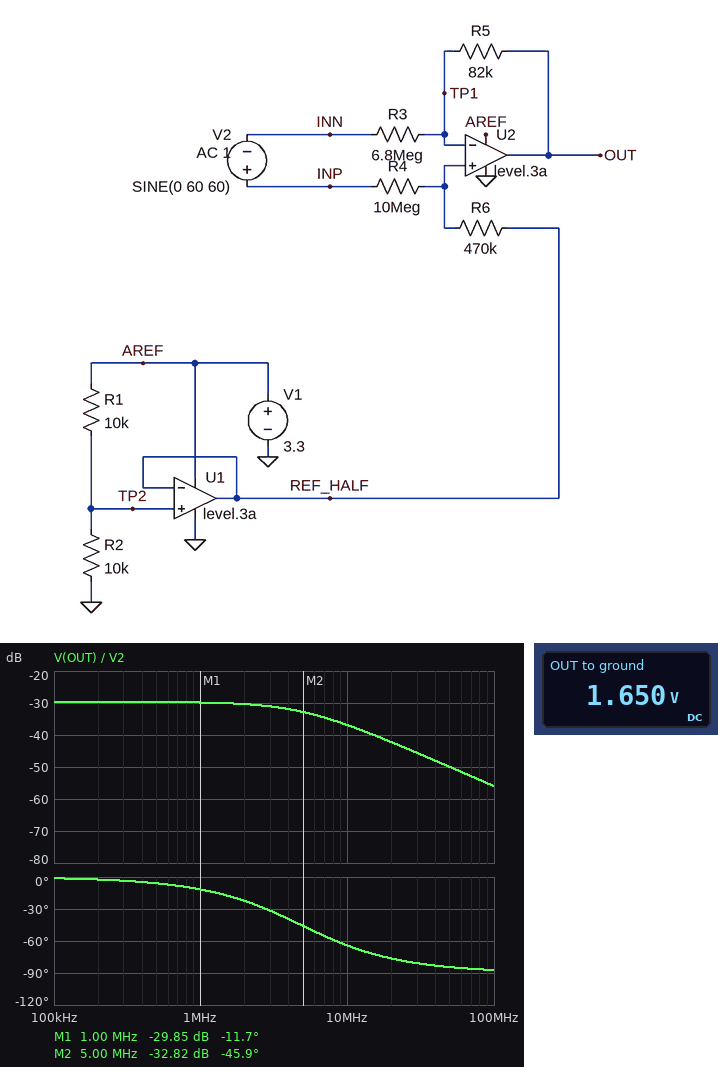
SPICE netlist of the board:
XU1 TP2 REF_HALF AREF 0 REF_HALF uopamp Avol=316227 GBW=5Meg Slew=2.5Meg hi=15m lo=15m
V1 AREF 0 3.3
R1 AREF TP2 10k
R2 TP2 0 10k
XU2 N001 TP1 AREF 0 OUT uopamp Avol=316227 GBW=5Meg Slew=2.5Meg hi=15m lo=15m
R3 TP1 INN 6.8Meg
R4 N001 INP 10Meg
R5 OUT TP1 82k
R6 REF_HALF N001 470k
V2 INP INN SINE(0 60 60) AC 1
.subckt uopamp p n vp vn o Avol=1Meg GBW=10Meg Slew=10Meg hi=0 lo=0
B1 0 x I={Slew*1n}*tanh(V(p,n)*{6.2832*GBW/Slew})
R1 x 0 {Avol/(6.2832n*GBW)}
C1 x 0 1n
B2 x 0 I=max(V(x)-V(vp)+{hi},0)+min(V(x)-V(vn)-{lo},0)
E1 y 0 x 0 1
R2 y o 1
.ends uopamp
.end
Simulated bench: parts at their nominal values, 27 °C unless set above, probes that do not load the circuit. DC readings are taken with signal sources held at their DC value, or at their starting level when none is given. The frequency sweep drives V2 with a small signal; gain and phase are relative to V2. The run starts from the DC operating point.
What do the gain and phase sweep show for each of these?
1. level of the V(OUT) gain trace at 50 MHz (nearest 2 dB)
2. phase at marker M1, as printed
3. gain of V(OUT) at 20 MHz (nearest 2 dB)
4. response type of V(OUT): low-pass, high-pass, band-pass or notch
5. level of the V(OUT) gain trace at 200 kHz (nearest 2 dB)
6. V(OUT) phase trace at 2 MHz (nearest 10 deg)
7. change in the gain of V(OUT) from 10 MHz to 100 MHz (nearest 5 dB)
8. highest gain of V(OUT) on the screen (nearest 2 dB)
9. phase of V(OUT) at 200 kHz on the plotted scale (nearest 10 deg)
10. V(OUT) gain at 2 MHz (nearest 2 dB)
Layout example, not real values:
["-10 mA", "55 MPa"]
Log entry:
["-50 dB", "-11.7 deg", "-42 dB", "low-pass", "-30 dB", "-20 deg", "-20 dB", "-30 dB", "0 deg", "-30 dB"]
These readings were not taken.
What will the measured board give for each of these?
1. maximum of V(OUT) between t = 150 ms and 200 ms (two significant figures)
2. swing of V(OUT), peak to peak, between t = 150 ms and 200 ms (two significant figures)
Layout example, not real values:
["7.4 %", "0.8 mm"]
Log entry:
["3.3 V", "3.3 V"]
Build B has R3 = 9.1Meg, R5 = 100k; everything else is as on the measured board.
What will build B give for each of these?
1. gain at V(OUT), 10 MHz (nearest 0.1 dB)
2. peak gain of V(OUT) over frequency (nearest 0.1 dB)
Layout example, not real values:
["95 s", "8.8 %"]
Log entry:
["-37.7 dB", "-30.5 dB"]
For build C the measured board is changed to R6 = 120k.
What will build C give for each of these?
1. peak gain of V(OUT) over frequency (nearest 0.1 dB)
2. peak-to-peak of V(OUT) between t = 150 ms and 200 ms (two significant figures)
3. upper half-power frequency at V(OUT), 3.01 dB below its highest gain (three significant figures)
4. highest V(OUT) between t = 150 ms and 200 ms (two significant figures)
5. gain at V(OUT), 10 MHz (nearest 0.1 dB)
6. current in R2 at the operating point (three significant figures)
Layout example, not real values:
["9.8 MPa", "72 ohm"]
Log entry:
["-38.4 dB", "1.4 V", "4.94 MHz", "2.4 V", "-45.5 dB", "165 µA"]
